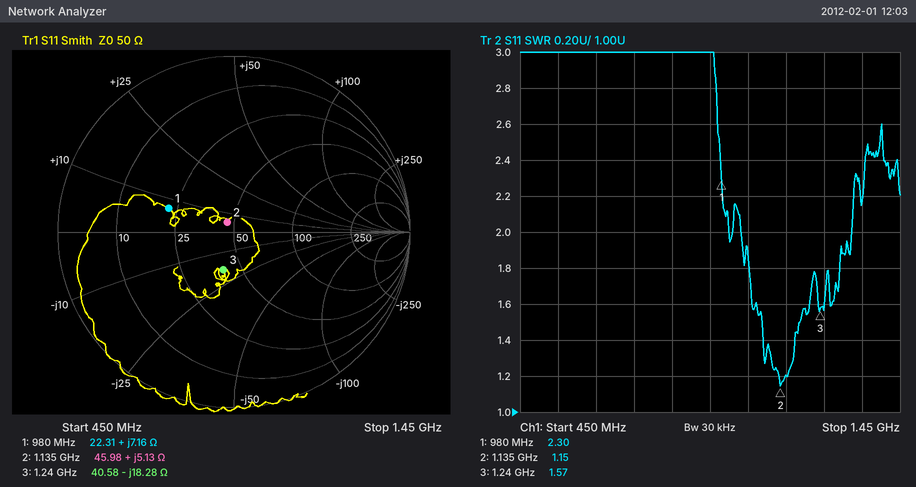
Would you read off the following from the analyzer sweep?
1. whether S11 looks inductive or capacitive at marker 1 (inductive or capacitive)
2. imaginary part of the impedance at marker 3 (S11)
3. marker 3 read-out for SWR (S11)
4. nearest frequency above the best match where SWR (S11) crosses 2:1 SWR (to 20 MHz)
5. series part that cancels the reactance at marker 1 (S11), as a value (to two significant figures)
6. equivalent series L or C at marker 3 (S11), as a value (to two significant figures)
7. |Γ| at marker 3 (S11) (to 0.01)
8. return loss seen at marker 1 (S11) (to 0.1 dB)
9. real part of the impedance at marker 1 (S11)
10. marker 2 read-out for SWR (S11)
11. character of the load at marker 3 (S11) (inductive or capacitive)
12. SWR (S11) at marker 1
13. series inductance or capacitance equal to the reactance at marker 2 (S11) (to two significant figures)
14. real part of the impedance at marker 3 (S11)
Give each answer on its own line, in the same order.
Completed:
inductive
-18.28 Ω
1.57
1.32 GHz
23 pF
7.0 pF
0.22
8.1 dB
22.31 Ω
1.15
capacitive
2.30
720 pH
40.58 Ω
